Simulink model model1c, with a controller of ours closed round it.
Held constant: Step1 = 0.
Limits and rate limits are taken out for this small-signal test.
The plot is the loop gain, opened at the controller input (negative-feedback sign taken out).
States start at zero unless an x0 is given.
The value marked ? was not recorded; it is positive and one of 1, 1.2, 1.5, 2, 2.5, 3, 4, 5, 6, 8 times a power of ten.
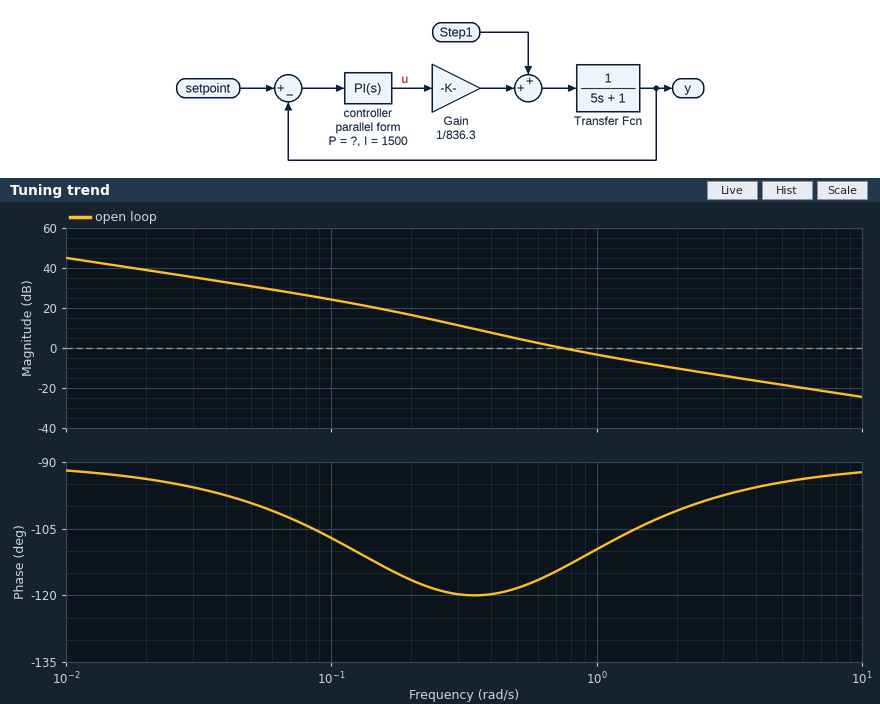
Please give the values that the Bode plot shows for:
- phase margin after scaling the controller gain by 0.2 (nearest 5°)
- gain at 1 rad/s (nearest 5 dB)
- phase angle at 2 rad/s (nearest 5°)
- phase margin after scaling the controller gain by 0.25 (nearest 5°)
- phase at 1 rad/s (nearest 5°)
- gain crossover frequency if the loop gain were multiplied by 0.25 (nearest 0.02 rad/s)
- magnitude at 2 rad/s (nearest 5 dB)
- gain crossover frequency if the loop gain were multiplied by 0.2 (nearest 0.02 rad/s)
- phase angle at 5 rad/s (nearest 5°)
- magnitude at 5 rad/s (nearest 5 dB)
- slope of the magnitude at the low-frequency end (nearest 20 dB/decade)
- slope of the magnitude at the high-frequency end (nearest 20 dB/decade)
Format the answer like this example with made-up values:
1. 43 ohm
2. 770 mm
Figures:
1. 60°
2. -5 dB
3. -100°
4. 60°
5. -110°
6. 0.28 rad/s
7. -10 dB
8. 0.24 rad/s
9. -95°
10. -20 dB
11. -20 dB/decade
12. -20 dB/decade
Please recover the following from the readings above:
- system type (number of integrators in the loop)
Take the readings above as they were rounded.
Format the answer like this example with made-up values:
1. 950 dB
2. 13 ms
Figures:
1. 1
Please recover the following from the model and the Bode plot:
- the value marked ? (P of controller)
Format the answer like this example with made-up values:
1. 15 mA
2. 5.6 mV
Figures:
1. 2500
